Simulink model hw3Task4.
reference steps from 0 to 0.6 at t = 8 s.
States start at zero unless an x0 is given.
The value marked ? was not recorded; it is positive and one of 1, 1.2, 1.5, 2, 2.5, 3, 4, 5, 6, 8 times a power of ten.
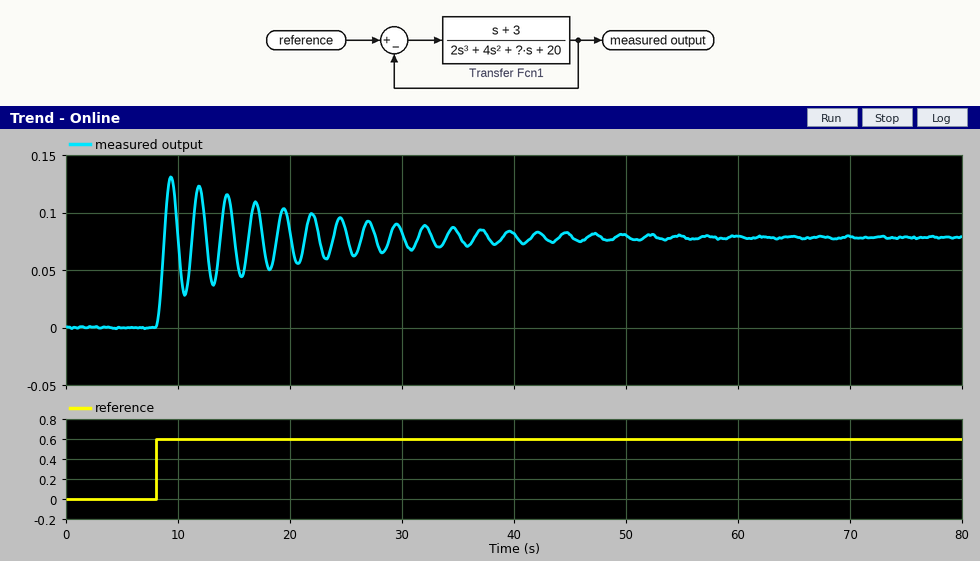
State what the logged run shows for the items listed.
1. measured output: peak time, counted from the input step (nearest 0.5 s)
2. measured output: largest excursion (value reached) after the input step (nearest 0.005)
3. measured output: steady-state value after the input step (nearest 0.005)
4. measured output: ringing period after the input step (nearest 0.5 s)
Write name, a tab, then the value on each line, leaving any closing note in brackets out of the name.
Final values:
measured output: peak time, counted from the input step	1.5 s
measured output: largest excursion (value reached) after the input step	0.130
measured output: steady-state value after the input step	0.080
measured output: ringing period after the input step	2.5 s
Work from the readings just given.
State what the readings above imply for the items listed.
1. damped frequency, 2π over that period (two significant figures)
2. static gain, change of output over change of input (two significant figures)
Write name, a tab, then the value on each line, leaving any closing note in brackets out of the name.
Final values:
damped frequency, 2π over that period	2.5 rad/s
static gain, change of output over change of input	0.13
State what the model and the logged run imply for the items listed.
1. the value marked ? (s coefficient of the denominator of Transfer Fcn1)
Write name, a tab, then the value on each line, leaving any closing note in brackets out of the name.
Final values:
the value marked ?	12
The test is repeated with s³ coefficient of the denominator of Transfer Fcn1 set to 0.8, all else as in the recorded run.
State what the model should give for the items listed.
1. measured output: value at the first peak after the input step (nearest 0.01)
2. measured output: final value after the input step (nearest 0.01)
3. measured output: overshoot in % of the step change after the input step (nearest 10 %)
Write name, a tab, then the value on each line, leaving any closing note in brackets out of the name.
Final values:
measured output: value at the first peak after the input step	0.10
measured output: final value after the input step	0.08
measured output: overshoot in % of the step change after the input step	30 %
